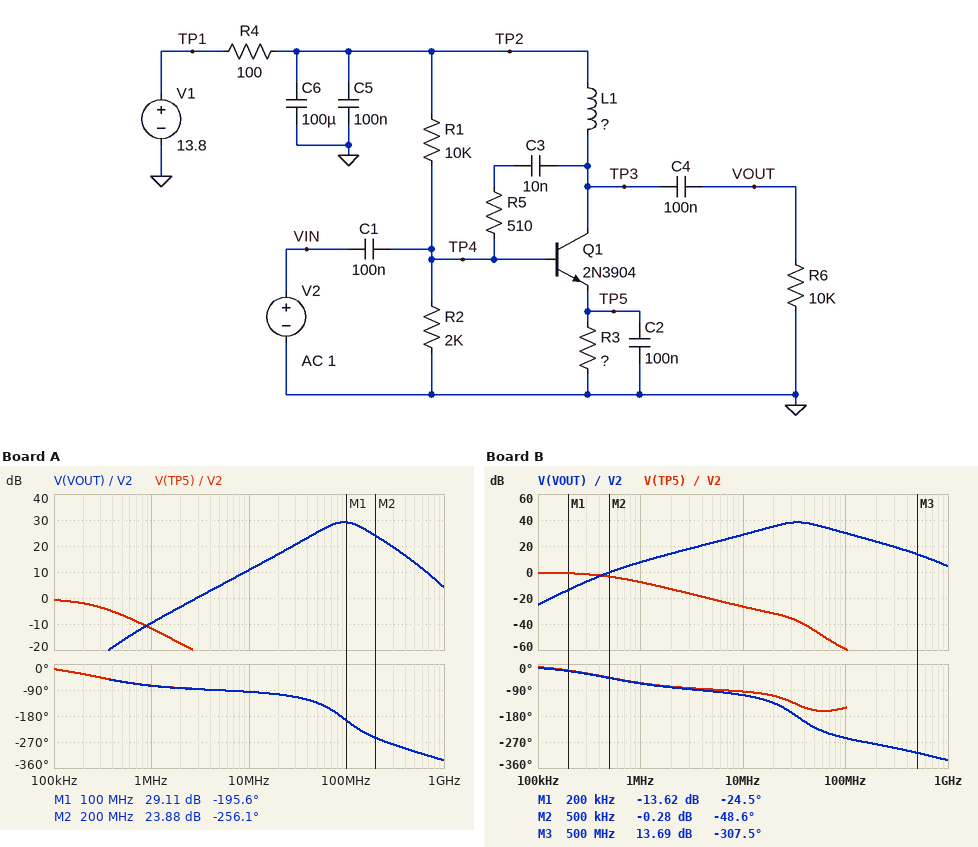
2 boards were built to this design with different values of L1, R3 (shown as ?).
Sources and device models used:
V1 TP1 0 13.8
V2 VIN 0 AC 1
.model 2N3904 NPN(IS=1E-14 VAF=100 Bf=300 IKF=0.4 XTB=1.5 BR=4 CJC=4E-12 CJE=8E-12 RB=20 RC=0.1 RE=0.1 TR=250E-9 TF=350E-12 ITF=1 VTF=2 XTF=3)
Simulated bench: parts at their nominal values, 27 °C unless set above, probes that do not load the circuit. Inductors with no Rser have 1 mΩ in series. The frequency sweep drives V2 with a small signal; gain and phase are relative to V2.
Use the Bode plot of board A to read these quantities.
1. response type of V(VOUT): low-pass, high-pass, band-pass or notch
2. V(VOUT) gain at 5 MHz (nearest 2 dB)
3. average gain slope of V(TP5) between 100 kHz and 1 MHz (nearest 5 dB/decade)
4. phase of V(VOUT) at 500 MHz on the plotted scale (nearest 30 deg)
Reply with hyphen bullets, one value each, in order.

- band-pass
- 4 dB
- -10 dB/decade
- -300 deg
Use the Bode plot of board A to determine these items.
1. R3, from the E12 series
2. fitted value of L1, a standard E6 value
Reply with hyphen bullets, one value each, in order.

- 330 Ω
- 330 nH
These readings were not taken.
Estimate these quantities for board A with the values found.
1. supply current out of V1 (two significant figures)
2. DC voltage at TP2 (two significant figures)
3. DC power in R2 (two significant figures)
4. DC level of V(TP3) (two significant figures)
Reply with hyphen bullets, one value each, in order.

- 5.6 mA
- 13 V
- 2.4 mW
- 13 V
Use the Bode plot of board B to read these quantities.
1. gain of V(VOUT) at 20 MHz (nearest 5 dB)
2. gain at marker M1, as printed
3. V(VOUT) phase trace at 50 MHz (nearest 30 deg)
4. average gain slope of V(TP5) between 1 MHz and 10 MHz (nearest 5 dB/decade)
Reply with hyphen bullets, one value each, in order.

- 35 dB
- -13.62 dB
- -210 deg
- -20 dB/decade
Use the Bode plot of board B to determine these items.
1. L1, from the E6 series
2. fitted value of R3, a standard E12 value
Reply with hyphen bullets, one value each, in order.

- 1.5 µH
- 180 Ω
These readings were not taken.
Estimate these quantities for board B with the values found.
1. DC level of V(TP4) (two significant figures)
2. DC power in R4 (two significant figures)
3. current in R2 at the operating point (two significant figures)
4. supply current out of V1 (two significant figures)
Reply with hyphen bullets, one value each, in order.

- 2.1 V
- 7.9 mW
- 1.1 mA
- 8.9 mA
